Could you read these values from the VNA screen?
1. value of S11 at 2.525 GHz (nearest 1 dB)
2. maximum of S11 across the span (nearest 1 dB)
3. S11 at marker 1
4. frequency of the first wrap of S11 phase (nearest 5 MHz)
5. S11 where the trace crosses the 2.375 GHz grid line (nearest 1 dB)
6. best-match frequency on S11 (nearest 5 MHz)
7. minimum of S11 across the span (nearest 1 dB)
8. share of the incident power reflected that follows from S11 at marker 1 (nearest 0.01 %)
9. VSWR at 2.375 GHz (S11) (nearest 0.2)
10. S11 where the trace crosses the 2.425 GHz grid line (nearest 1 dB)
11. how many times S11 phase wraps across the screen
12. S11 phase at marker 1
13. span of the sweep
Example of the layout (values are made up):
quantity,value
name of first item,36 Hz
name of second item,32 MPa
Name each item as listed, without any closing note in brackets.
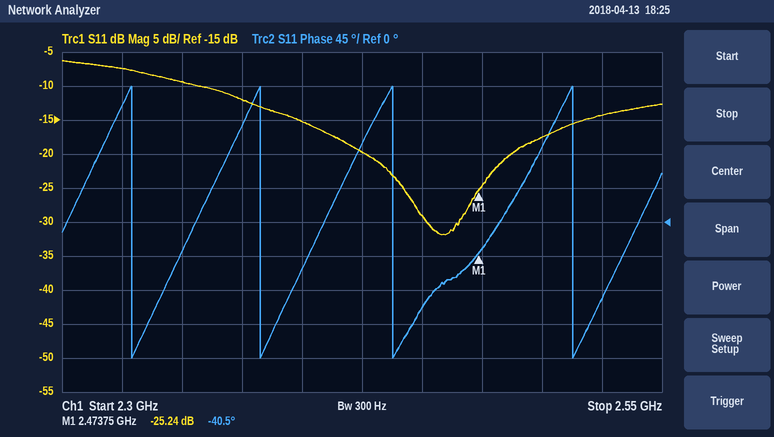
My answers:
quantity,value
value of S11 at 2.525 GHz,-14 dB
maximum of S11 across the span,-6 dB
S11 at marker 1,-25.24 dB
frequency of the first wrap of S11 phase,2.330 GHz
S11 where the trace crosses the 2.375 GHz grid line,-12 dB
best-match frequency on S11,2.460 GHz
minimum of S11 across the span,-32 dB
share of the incident power reflected that follows from S11 at marker 1,0.30 %
VSWR at 2.375 GHz (S11),1.6
S11 where the trace crosses the 2.425 GHz grid line,-20 dB
how many times S11 phase wraps across the screen,4
S11 phase at marker 1,-40.5°
span of the sweep,250 MHz
